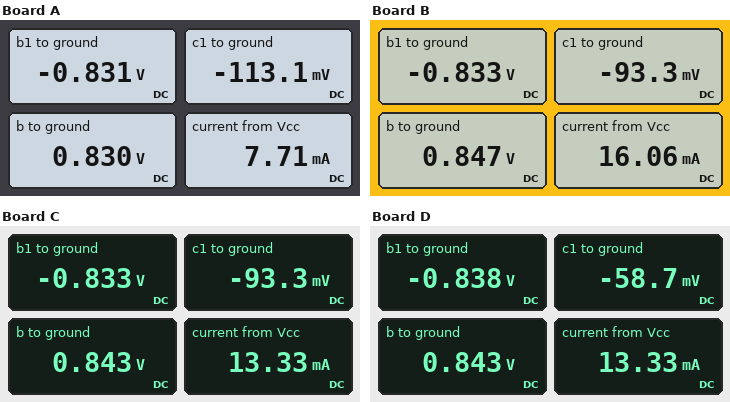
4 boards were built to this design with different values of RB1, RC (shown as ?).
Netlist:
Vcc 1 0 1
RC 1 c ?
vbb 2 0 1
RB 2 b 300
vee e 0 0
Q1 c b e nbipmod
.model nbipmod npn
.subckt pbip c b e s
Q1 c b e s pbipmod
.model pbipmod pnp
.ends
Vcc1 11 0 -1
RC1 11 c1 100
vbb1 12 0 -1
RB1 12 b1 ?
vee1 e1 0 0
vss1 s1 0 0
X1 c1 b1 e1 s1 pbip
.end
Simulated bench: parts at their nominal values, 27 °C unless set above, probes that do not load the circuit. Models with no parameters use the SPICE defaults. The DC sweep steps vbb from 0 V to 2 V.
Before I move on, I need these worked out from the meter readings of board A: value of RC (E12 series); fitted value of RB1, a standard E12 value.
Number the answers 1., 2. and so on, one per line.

1. 120 Ω
2. 820 Ω
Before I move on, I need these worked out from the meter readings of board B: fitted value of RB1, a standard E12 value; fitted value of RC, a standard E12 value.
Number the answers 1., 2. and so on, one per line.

1. 470 Ω
2. 56 Ω
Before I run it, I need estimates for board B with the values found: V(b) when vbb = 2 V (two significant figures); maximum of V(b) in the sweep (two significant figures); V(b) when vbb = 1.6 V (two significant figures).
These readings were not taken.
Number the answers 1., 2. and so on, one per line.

1. 860 mV
2. 860 mV
3. 850 mV
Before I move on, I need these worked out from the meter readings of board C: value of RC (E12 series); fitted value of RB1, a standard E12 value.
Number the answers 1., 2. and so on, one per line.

1. 68 Ω
2. 470 Ω
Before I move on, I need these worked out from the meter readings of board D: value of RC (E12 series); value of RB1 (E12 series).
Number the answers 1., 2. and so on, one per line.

1. 68 Ω
2. 120 Ω
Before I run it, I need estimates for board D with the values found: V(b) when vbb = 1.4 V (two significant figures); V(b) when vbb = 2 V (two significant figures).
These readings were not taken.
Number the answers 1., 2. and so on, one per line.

1. 850 mV
2. 850 mV
